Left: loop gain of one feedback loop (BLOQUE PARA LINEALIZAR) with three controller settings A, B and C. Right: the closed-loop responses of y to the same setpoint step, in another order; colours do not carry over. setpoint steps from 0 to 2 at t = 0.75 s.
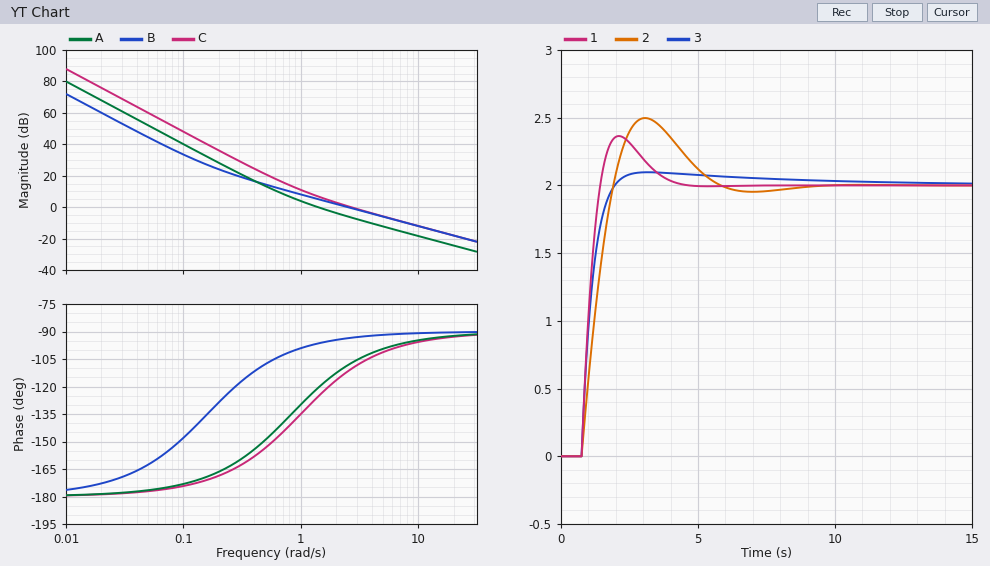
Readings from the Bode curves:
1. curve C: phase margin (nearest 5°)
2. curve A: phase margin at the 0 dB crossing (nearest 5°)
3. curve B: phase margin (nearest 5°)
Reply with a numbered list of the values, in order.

1. 70°
2. 60°
3. 85°
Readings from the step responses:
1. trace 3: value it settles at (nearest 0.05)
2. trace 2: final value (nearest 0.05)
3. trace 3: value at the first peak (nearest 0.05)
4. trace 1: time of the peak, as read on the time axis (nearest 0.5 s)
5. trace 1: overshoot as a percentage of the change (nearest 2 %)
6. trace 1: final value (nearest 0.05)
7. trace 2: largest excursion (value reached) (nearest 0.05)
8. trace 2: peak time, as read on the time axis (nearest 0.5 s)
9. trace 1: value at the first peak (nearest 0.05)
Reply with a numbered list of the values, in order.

1. 2.00
2. 2.00
3. 2.10
4. 2.0 s
5. 18 %
6. 2.00
7. 2.50
8. 3.0 s
9. 2.35
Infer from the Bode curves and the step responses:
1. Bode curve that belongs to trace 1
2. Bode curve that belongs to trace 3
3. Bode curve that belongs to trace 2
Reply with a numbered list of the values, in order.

1. C
2. B
3. A
